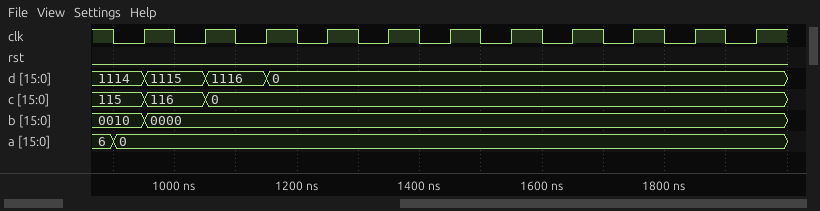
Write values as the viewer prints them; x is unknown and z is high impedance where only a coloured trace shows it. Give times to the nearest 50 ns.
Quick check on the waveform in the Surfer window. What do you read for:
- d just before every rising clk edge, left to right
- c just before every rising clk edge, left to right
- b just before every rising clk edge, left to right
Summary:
1114, 1115, 1116, 0, 0, 0, 0, 0, 0, 0, 0
115, 116, 0, 0, 0, 0, 0, 0, 0, 0, 0
0010, 0000, 0000, 0000, 0000, 0000, 0000, 0000, 0000, 0000, 0000
